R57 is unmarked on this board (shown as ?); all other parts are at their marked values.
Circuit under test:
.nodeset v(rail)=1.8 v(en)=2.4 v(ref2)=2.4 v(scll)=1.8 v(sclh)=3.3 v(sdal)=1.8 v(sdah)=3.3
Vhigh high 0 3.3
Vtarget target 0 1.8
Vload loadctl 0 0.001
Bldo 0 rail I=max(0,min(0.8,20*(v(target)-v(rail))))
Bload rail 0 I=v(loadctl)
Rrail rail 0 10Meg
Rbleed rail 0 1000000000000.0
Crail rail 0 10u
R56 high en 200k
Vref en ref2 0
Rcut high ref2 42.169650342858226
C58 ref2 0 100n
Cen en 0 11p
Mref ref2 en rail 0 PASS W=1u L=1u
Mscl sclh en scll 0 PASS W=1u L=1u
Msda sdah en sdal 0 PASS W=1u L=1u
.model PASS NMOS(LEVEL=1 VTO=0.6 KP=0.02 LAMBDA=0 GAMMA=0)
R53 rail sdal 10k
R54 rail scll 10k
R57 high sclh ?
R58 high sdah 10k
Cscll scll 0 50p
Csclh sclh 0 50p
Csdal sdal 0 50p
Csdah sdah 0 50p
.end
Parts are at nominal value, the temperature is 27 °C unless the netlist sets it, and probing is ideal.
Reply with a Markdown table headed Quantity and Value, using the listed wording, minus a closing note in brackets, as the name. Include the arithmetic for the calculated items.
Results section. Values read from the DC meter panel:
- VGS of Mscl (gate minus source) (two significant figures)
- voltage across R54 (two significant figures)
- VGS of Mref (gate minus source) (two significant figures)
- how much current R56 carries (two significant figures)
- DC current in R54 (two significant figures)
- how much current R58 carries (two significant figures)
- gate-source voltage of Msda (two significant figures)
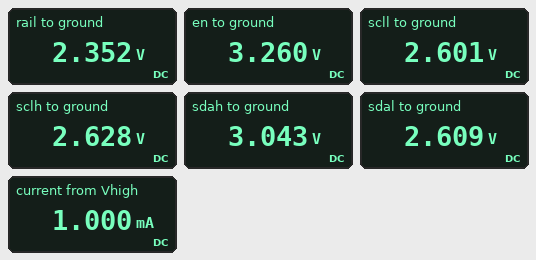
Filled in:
| Quantity | Value |
|---|---|
| VGS of Mscl (gate minus source) | 3.26 V - 2.601 V = 660 mV |
| voltage across R54 | 2.601 V - 2.352 V = 250 mV |
| VGS of Mref (gate minus source) | 3.26 V - 2.352 V = 910 mV |
| how much current R56 carries | (3.3 V - 3.26 V) / 200 kΩ = 200 nA |
| DC current in R54 | (2.601 V - 2.352 V) / 10 kΩ = 25 µA |
| how much current R58 carries | (3.3 V - 3.043 V) / 10 kΩ = 26 µA |
| gate-source voltage of Msda | 3.26 V - 2.609 V = 650 mV |
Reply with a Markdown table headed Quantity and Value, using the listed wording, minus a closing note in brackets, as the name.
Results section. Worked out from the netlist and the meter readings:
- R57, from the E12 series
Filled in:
| Quantity | Value |
|---|---|
| R57, from the E12 series | 27 kΩ |
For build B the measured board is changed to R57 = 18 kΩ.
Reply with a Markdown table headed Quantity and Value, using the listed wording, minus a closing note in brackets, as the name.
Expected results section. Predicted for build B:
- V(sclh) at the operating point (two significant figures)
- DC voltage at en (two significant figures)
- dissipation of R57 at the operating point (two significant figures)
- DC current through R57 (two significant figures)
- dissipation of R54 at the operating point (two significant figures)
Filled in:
| Quantity | Value |
|---|---|
| V(sclh) at the operating point | 2.8 V |
| DC voltage at en | 3.3 V |
| dissipation of R57 at the operating point | 12 µW |
| DC current through R57 | 26 µA |
| dissipation of R54 at the operating point | 6.6 µW |
